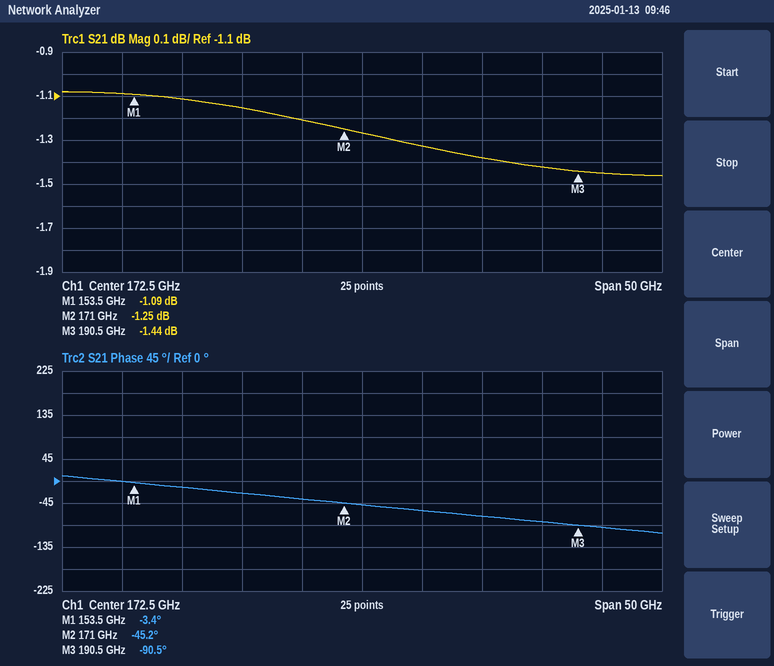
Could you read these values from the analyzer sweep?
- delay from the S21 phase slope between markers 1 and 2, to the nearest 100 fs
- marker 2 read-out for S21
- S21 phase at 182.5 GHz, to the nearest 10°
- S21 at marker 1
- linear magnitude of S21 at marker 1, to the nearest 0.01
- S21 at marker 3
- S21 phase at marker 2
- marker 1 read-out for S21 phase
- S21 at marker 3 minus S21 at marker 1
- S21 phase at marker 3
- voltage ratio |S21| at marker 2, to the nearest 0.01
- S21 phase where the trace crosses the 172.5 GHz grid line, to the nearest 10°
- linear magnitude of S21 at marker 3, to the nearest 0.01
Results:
6.6 ps
-1.25 dB
-70°
-1.09 dB
0.88
-1.44 dB
-45.2°
-3.4°
-0.35 dB
-90.5°
0.87
-50°
0.85
